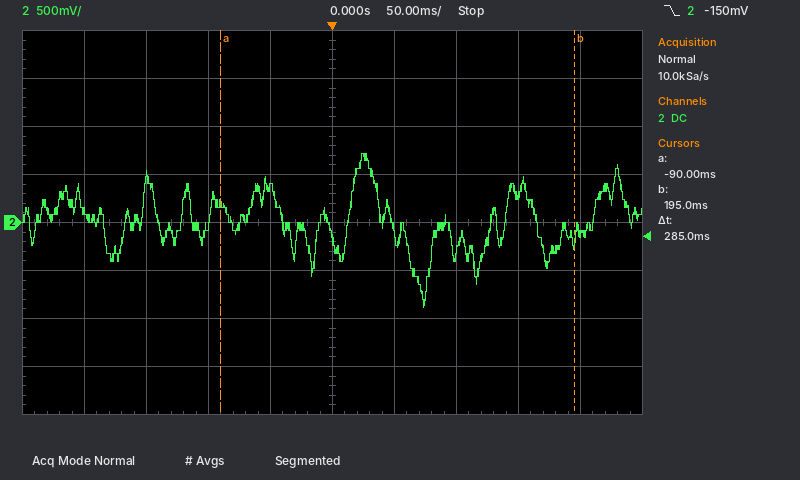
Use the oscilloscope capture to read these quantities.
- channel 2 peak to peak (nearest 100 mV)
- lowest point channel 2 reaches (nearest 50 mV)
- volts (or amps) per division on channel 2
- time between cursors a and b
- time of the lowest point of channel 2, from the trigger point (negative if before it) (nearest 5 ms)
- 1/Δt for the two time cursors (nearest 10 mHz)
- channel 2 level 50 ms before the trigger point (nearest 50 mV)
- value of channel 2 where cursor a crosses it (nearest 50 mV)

1.60 V
-900 mV
500 mV
285 ms
+75 ms
3.51 Hz
350 mV
200 mV
